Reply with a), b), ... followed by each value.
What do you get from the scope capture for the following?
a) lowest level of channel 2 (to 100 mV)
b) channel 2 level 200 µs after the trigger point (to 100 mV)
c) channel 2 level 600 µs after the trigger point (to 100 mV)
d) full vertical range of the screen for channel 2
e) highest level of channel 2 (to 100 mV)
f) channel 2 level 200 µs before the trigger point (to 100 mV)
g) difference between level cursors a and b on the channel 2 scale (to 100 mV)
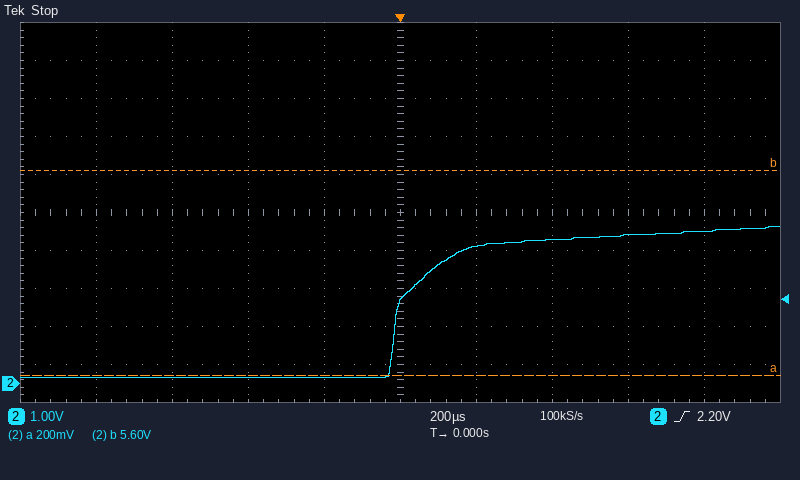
a) 200 mV
b) 3.6 V
c) 3.9 V
d) 10 V
e) 4.1 V
f) 200 mV
g) 5.4 V
